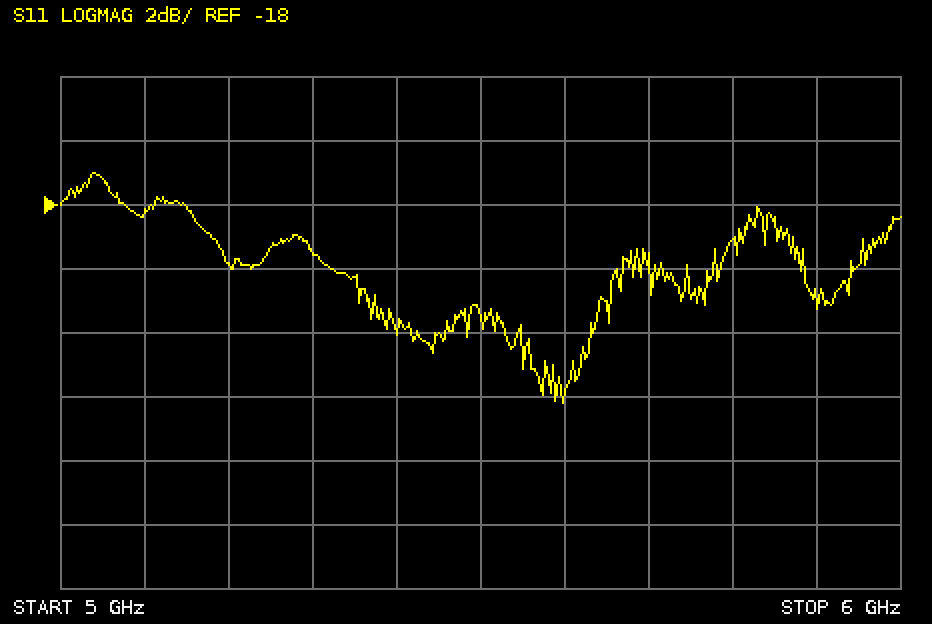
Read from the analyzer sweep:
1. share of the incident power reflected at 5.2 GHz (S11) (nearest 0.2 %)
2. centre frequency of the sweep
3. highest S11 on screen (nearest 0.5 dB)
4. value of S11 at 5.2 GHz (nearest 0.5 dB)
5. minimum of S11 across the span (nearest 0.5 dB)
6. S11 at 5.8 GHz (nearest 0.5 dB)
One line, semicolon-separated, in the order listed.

1.0 %; 5.5 GHz; -17.0 dB; -20.0 dB; -24.0 dB; -19.0 dB
